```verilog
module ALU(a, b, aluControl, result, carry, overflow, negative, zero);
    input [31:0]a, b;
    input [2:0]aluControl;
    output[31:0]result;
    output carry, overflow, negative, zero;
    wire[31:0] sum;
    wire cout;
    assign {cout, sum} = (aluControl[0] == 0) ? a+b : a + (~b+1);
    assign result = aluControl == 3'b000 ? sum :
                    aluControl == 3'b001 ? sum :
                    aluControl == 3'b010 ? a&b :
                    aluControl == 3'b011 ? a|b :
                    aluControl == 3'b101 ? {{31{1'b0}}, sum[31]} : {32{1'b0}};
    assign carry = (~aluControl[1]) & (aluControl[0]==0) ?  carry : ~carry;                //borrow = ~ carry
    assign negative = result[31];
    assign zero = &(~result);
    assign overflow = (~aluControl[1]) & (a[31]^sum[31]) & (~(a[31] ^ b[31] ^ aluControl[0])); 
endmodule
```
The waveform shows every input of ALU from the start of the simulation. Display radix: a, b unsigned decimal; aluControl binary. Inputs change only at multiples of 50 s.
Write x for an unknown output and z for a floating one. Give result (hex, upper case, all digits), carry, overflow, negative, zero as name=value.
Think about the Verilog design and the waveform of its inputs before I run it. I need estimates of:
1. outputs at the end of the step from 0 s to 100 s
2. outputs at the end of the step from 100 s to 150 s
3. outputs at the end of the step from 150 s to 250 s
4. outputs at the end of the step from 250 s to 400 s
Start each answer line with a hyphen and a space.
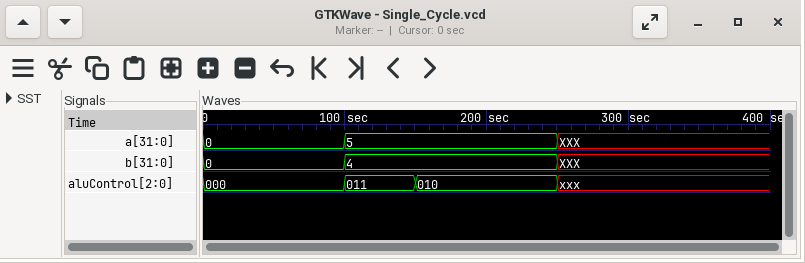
- result=00000000, carry=z, overflow=0, negative=0, zero=1
- result=00000005, carry=z, overflow=0, negative=0, zero=0
- result=00000004, carry=z, overflow=0, negative=0, zero=0
- result=x, carry=z, overflow=x, negative=x, zero=x
